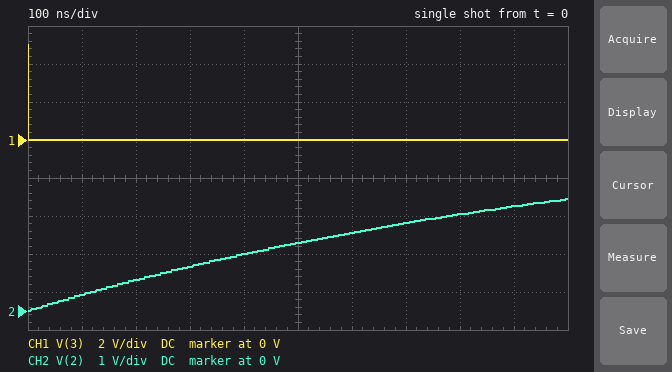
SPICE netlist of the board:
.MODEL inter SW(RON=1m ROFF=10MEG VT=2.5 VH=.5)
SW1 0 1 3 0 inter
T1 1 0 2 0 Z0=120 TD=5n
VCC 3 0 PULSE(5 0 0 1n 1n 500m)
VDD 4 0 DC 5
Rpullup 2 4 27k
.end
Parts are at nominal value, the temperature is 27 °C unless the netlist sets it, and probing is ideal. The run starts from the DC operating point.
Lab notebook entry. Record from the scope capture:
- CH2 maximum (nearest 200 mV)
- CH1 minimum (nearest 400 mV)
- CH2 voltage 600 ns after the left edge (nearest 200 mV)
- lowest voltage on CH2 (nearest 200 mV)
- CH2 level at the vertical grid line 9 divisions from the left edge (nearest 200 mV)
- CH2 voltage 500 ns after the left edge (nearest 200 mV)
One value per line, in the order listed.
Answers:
3.0 V
0 V
2.0 V
0 V
2.8 V
1.8 V
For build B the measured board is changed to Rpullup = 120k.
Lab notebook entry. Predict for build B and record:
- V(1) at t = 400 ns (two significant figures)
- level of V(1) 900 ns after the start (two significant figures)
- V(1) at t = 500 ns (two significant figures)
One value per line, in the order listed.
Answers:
380 mV
820 mV
470 mV
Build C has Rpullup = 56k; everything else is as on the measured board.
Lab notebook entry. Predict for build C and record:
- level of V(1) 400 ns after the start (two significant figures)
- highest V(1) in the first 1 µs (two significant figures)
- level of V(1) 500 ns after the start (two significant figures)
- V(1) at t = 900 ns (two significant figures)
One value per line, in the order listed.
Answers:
780 mV
1.7 V
960 mV
1.6 V
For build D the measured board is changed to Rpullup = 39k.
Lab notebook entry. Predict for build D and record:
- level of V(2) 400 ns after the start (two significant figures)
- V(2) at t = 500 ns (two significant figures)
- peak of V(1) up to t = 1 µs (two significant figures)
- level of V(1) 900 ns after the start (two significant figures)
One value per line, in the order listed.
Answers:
1.1 V
1.3 V
2.3 V
2.1 V
